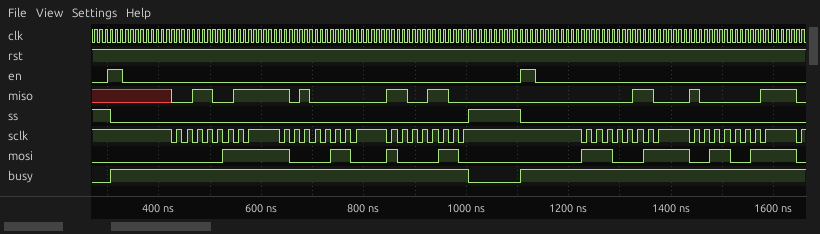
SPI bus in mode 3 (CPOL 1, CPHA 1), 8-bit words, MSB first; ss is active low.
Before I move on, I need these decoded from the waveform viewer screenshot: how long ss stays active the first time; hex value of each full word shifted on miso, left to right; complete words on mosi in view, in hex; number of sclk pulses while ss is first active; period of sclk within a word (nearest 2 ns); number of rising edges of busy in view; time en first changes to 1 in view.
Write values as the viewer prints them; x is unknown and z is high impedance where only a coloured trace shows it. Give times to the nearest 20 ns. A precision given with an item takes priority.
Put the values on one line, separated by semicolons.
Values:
700 ns; 33, A0, CC, 06, 81; 07, 86, 86, E3, 33; 24; 20 ns; 2; 300 ns
